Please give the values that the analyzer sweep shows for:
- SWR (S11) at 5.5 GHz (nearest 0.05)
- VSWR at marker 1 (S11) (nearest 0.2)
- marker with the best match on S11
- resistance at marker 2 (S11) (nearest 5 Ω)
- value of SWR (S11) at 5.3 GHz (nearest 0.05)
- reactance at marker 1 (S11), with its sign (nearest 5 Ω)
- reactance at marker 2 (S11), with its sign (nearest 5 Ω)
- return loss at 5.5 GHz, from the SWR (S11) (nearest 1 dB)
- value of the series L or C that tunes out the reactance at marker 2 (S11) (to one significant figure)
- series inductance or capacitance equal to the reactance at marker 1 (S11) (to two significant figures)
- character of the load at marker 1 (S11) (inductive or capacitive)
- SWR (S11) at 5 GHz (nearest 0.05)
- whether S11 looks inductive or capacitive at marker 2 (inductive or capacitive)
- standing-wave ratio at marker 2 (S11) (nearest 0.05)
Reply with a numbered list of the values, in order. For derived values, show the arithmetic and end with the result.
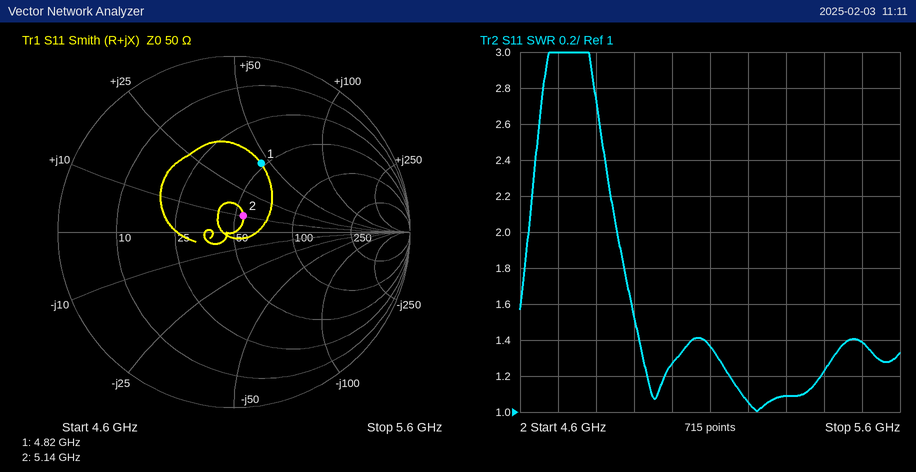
1. 1.40
2. 2.4
3. marker 2
4. 55 Ω
5. 1.10
6. +45 Ω
7. +10 Ω
8. −20 log10((1.4 − 1)/(1.4 + 1)) ≈ 16 dB
9. C = 1/(2π × 5.14 GHz × 10 Ω) ≈ 3 pF
10. L = 45 Ω/(2π × 4.82 GHz) ≈ 1.5 nH
11. inductive
12. 1.25
13. inductive
14. 1.25
